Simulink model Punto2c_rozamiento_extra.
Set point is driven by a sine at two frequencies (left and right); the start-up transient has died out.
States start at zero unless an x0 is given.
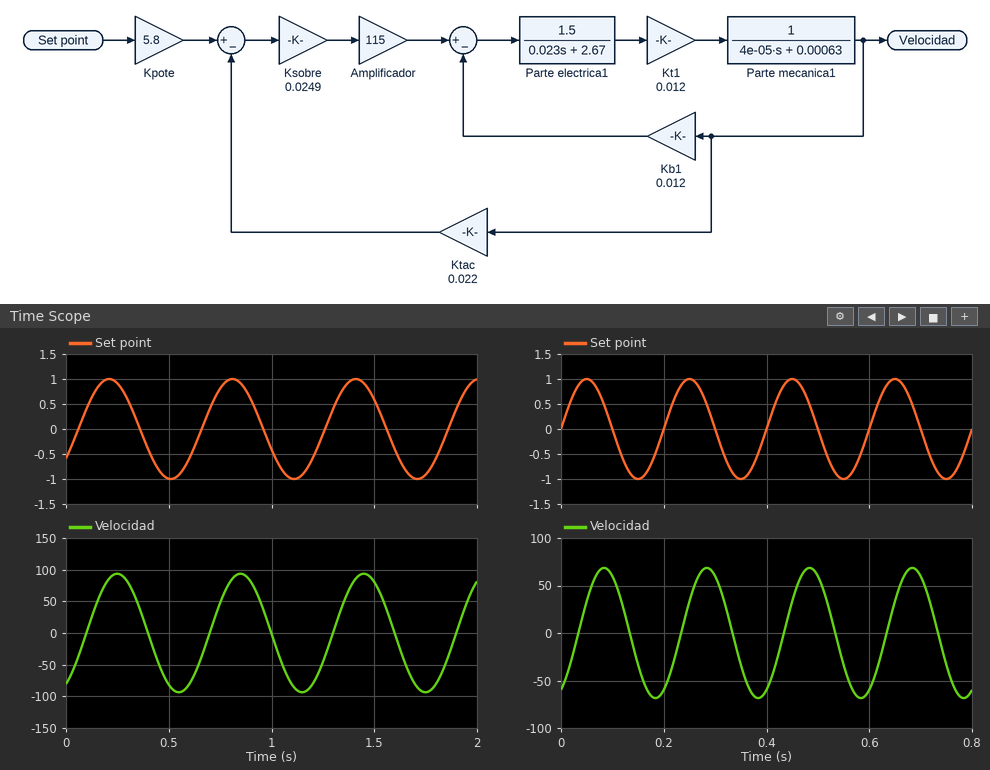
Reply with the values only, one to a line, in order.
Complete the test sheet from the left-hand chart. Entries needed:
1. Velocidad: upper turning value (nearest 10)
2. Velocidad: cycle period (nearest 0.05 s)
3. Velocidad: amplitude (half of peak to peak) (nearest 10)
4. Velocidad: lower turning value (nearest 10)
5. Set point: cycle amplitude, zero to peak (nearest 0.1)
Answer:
90
0.60 s
90
-90
1.0
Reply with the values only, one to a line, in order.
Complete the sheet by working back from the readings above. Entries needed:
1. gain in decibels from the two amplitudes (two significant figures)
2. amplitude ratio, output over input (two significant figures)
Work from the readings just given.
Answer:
39 dB
90
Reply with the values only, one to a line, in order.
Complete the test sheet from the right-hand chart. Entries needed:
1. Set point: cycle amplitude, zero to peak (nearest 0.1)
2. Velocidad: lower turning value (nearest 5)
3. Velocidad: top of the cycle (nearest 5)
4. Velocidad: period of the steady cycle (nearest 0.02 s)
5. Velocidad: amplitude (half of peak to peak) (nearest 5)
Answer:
1.0
-70
70
0.20 s
70
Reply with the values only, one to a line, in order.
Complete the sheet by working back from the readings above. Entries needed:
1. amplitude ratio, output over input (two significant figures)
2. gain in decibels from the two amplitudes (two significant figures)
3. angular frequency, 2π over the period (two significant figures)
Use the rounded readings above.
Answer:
70
37 dB
31 rad/s
